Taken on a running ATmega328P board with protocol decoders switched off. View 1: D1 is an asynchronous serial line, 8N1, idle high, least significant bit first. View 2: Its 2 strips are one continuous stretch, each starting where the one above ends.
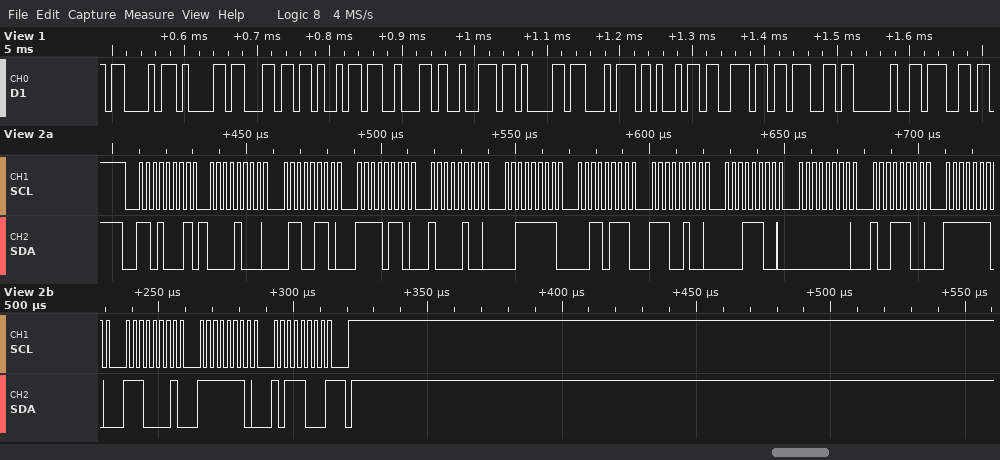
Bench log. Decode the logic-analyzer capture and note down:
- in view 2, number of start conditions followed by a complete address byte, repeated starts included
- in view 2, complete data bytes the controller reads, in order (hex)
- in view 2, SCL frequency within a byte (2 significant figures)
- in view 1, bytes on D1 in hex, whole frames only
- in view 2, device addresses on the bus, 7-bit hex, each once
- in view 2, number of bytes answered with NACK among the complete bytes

1
08 66 F6 84 3F 37 E4 1C 00 9C FE E1 FE B8
400 kHz
43 61 6C 69 62 72 61 74 69 6E 67 20 67
0x68
1
